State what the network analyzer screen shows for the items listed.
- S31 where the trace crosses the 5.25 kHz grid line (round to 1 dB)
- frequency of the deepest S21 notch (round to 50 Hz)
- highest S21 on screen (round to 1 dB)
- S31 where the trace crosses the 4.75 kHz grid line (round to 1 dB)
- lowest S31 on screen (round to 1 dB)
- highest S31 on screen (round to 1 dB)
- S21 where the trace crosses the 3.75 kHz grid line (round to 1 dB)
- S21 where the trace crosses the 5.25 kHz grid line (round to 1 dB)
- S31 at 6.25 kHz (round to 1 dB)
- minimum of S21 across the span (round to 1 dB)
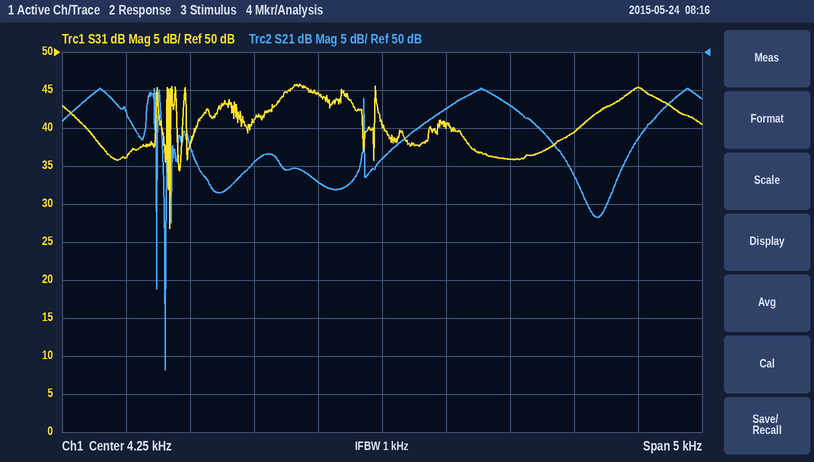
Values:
36 dB
2.55 kHz
45 dB
40 dB
27 dB
46 dB
33 dB
43 dB
45 dB
8 dB
